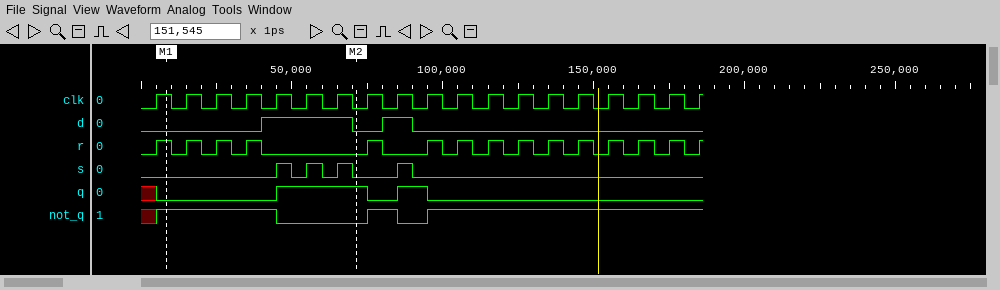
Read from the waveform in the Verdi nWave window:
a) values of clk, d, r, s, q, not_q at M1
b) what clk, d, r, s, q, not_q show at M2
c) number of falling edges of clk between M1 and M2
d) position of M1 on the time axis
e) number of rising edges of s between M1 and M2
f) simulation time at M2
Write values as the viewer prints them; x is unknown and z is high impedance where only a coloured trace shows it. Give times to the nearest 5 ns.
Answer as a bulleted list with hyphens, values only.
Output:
- clk=1, d=0, r=1, s=0, q=0, not_q=1
- clk=0, d=0, r=0, s=0, q=1, not_q=0
- 7
- 10 ns
- 3
- 70 ns
